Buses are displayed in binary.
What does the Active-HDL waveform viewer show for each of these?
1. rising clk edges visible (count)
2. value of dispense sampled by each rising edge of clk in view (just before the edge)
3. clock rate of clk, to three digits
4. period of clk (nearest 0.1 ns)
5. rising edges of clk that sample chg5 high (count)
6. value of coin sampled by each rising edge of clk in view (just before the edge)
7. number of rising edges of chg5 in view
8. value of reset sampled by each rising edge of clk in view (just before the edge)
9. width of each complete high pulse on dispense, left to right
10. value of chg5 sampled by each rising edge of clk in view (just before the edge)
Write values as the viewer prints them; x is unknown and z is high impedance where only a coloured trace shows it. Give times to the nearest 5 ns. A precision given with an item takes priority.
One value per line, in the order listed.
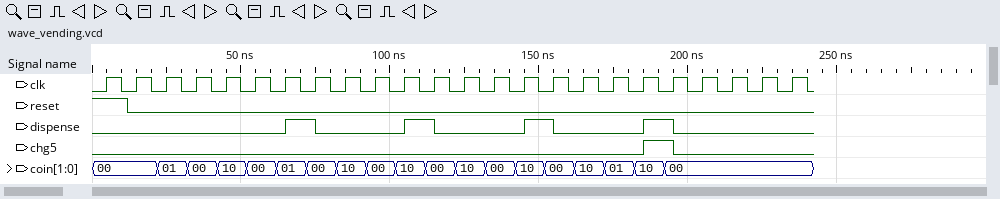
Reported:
24
0 0 0 0 0 0 0 1 0 0 0 1 0 0 0 1 0 0 0 1 0 0 0 0
100 MHz
10 ns
1
00, 00, 01, 00, 10, 00, 01, 00, 10, 00, 10, 00, 10, 00, 10, 00, 10, 01, 10, 00, 00, 00, 00, 00
1
1 0 0 0 0 0 0 0 0 0 0 0 0 0 0 0 0 0 0 0 0 0 0 0
10 ns, 10 ns, 10 ns, 10 ns
0 0 0 0 0 0 0 0 0 0 0 0 0 0 0 0 0 0 0 1 0 0 0 0
